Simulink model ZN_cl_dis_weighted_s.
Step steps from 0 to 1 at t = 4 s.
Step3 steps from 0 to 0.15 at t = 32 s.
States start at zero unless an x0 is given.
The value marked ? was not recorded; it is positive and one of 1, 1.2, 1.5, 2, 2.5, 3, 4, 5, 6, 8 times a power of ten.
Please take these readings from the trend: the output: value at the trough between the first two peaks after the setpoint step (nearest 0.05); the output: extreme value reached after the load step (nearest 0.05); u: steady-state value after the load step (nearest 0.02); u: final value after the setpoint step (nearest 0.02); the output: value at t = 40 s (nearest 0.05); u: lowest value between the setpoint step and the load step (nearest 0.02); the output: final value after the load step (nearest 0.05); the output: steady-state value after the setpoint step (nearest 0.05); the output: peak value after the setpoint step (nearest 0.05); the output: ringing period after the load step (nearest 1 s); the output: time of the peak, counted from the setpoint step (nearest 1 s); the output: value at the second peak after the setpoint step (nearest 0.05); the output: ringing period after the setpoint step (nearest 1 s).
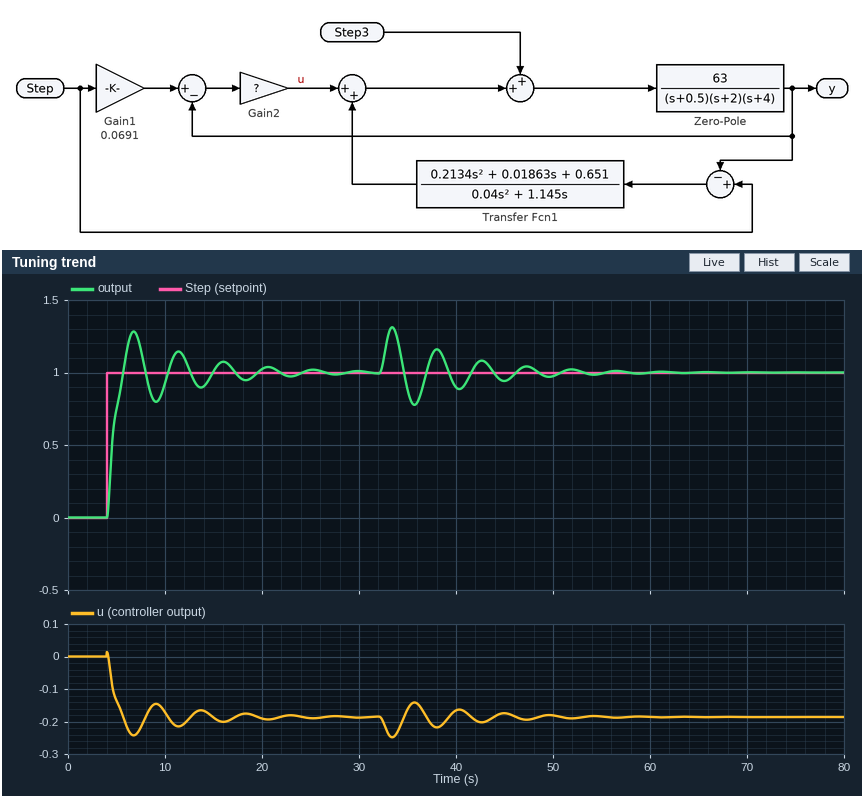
0.80
1.30
-0.18
-0.18
0.90
-0.24
1.00
1.00
1.30
5 s
3 s
1.15
5 s
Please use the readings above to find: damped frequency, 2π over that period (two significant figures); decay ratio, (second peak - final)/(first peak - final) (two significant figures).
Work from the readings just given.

1.3 rad/s
0.50
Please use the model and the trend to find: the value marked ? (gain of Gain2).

0.2
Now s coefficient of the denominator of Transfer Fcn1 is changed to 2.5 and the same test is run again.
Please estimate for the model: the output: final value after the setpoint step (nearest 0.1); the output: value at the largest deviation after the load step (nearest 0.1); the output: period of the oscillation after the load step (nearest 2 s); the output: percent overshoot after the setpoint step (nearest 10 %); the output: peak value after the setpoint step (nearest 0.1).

1.0
1.4
6 s
20 %
1.2
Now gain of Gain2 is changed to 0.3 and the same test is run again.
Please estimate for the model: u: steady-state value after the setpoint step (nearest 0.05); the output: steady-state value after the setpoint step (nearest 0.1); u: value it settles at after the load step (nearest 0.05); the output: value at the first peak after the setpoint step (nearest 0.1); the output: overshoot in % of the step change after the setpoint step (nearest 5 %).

-0.30
1.0
-0.30
1.2
20 %
